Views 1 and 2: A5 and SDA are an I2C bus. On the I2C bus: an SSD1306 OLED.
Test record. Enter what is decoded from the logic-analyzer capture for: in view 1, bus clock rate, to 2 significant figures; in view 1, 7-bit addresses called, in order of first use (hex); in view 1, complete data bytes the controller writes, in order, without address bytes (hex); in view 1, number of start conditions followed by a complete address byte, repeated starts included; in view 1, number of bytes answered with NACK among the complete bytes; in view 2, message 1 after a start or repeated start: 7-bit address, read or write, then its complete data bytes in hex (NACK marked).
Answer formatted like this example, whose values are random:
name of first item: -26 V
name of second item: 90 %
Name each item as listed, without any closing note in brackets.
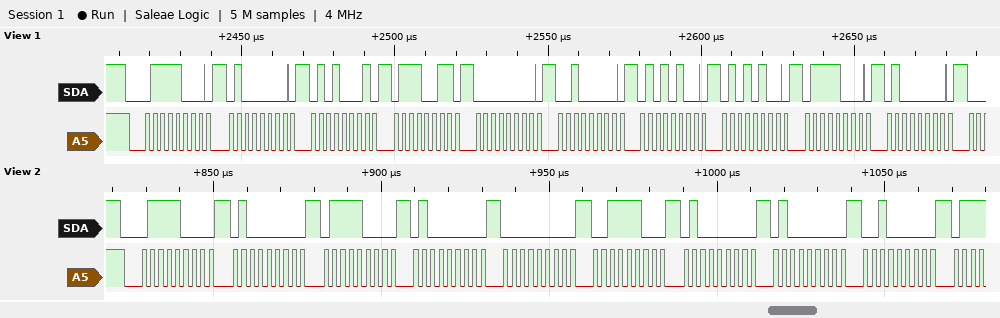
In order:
in view 1, bus clock rate, to 2 significant figures: 400 kHz
in view 1, 7-bit addresses called, in order of first use: 0x3C
in view 1, complete data bytes the controller writes, in order, without address bytes: 40 51 73 00 20 54 54 78 40
in view 1, number of start conditions followed by a complete address byte, repeated starts included: 1
in view 1, number of bytes answered with NACK among the complete bytes: 0
in view 2, message 1 after a start or repeated start: 7-bit address, read or write, then its complete data bytes in hex: 0x3C write: 40 78 40 00 3C 40 40 20
